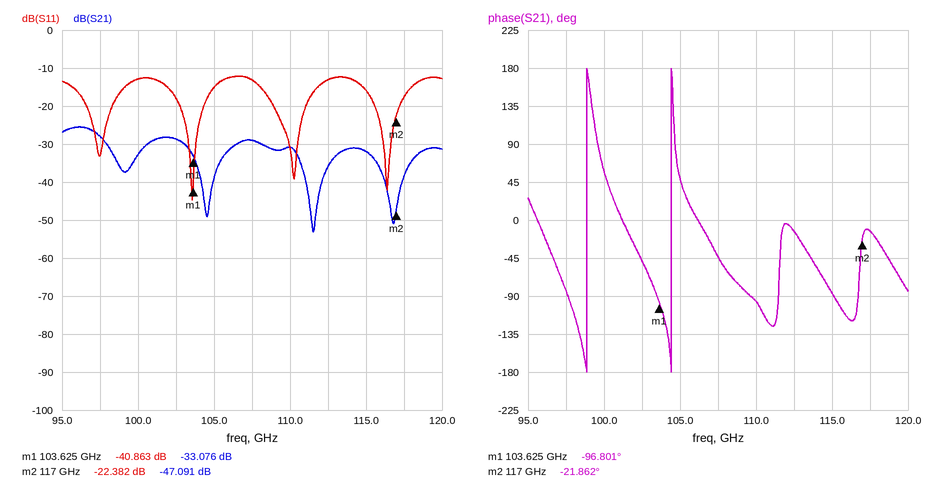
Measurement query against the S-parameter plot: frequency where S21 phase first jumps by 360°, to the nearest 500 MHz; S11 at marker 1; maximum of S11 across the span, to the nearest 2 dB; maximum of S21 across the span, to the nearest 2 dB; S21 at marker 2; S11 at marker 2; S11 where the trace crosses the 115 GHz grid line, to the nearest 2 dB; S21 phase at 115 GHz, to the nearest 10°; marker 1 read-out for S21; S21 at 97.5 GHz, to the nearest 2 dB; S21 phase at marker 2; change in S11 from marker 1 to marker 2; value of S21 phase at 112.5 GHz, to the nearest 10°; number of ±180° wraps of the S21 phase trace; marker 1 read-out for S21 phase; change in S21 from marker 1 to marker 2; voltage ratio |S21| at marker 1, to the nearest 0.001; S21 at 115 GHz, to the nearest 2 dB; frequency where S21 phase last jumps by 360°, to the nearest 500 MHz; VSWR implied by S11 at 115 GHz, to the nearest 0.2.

99.0 GHz
-40.863 dB
-12 dB
-26 dB
-47.091 dB
-22.382 dB
-16 dB
-90°
-33.076 dB
-28 dB
-21.862°
18.481 dB
-10°
2
-96.801°
-14.015 dB
0.022
-32 dB
104.5 GHz
1.4
